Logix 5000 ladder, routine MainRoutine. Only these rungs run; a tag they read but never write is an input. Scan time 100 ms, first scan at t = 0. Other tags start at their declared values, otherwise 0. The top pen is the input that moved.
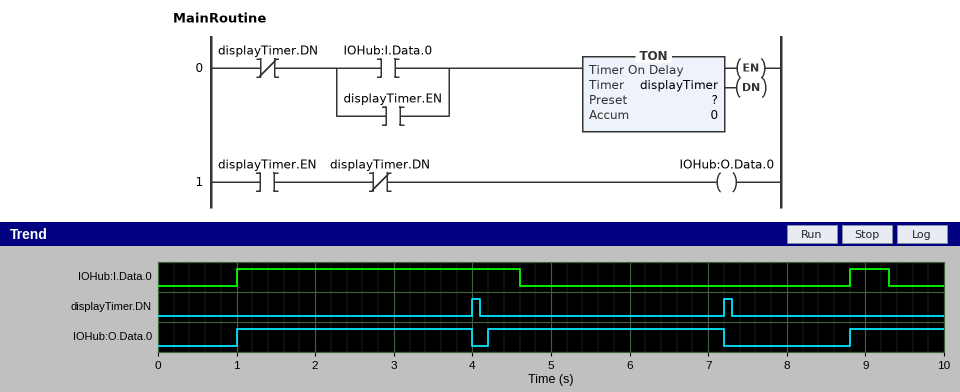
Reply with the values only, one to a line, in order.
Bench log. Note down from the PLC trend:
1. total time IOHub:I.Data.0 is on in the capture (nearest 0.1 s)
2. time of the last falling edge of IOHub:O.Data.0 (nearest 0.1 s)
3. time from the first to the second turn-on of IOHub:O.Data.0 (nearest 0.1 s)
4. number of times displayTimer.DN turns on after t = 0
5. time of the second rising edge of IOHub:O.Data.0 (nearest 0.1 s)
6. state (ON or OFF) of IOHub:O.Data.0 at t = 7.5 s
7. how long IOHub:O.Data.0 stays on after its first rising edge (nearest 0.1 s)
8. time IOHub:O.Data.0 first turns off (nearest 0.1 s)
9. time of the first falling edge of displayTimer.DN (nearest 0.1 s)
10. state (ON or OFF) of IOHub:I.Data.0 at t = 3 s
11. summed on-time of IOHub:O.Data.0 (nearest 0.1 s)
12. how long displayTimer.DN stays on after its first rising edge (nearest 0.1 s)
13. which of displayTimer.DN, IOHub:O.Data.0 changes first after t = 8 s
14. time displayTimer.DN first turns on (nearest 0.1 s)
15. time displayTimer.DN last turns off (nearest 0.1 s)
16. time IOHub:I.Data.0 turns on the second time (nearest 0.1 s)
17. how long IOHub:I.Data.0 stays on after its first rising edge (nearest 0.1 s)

4.1 s
7.2 s
3.2 s
2
4.2 s
OFF
3.0 s
4.0 s
4.1 s
ON
7.2 s
0.1 s
IOHub:O.Data.0
4.0 s
7.3 s
8.8 s
3.6 s
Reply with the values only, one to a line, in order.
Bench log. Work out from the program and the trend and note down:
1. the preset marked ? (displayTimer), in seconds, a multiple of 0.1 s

3.0 s
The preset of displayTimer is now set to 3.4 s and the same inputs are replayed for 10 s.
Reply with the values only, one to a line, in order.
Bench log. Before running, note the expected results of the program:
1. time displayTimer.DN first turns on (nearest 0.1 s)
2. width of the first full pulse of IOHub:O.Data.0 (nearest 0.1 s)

4.4 s
3.4 s
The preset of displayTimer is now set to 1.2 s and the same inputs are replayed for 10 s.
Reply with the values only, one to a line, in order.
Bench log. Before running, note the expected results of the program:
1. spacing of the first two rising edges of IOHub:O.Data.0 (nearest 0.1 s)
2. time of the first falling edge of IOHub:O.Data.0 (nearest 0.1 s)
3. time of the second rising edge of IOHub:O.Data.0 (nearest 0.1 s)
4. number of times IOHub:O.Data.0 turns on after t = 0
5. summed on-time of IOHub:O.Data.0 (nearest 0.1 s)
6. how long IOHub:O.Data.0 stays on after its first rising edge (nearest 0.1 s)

1.4 s
2.2 s
2.4 s
4
4.8 s
1.2 s
